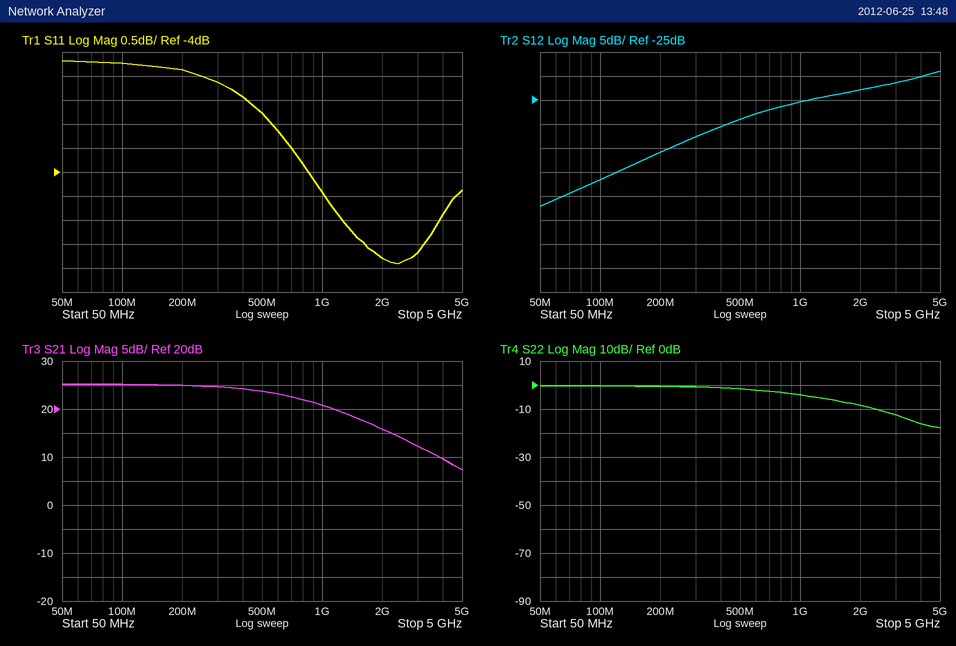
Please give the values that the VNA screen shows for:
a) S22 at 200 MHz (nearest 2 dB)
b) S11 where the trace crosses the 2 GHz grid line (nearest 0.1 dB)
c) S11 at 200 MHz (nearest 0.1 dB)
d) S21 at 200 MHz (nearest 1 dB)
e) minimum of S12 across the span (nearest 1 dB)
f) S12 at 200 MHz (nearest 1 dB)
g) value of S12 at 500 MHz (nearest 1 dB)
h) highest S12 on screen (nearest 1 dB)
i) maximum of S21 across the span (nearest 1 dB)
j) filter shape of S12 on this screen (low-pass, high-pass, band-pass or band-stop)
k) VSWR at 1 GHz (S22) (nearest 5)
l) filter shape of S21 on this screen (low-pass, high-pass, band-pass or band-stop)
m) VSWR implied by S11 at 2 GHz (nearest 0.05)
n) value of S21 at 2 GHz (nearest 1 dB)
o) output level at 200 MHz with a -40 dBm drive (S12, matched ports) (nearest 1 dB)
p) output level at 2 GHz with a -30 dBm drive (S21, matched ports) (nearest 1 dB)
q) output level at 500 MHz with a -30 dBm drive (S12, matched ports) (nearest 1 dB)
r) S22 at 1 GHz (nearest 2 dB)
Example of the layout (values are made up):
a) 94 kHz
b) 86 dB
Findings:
a) 0 dB
b) -5.8 dB
c) -1.9 dB
d) 25 dB
e) -47 dB
f) -36 dB
g) -29 dB
h) -19 dB
i) 25 dB
j) high-pass
k) 5
l) low-pass
m) 3.10
n) 16 dB
o) -76 dBm
p) -14 dBm
q) -59 dBm
r) -4 dB
